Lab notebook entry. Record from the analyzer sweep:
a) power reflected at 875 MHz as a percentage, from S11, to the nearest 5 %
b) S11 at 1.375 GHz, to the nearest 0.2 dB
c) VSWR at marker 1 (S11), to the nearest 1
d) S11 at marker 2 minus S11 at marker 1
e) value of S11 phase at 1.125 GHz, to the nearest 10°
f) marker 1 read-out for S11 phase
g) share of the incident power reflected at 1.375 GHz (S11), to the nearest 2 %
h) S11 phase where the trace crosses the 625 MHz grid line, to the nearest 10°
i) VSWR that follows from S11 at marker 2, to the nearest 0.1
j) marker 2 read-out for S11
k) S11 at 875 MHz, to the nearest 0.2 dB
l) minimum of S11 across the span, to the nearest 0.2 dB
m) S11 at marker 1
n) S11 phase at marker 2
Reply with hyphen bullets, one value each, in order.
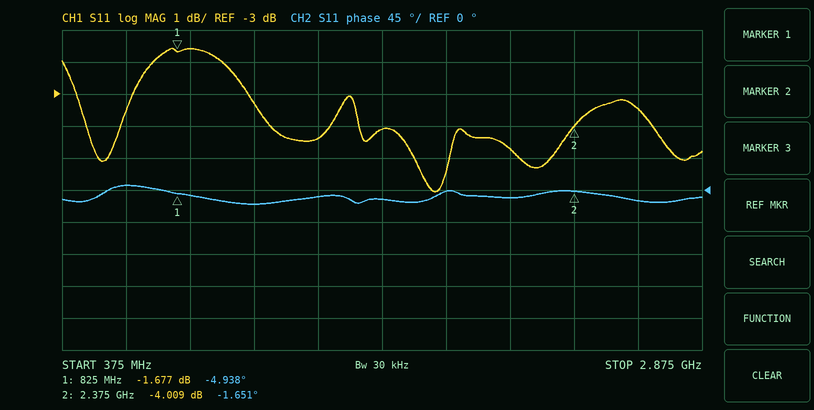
- 70 %
- -4.4 dB
- 10
- -2.332 dB
- -20°
- -4.938°
- 36 %
- 10°
- 4.4
- -4.009 dB
- -1.6 dB
- -6.0 dB
- -1.677 dB
- -1.651°
